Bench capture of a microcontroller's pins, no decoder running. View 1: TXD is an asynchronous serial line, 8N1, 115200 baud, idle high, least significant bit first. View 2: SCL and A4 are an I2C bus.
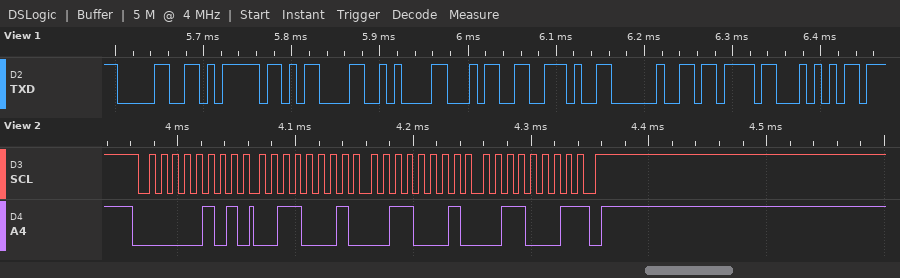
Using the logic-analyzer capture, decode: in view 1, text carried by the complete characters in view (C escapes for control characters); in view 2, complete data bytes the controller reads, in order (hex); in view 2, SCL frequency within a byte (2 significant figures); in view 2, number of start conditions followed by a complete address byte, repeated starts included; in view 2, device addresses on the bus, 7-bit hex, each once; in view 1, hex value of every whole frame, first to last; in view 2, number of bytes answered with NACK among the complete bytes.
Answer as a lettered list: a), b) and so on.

a) "0}\r\n4. {T"
b) 31 31 31
c) 100 kHz
d) 1
e) 0x02
f) 30 7D 0D 0A 34 2E 20 7B 54
g) 1
